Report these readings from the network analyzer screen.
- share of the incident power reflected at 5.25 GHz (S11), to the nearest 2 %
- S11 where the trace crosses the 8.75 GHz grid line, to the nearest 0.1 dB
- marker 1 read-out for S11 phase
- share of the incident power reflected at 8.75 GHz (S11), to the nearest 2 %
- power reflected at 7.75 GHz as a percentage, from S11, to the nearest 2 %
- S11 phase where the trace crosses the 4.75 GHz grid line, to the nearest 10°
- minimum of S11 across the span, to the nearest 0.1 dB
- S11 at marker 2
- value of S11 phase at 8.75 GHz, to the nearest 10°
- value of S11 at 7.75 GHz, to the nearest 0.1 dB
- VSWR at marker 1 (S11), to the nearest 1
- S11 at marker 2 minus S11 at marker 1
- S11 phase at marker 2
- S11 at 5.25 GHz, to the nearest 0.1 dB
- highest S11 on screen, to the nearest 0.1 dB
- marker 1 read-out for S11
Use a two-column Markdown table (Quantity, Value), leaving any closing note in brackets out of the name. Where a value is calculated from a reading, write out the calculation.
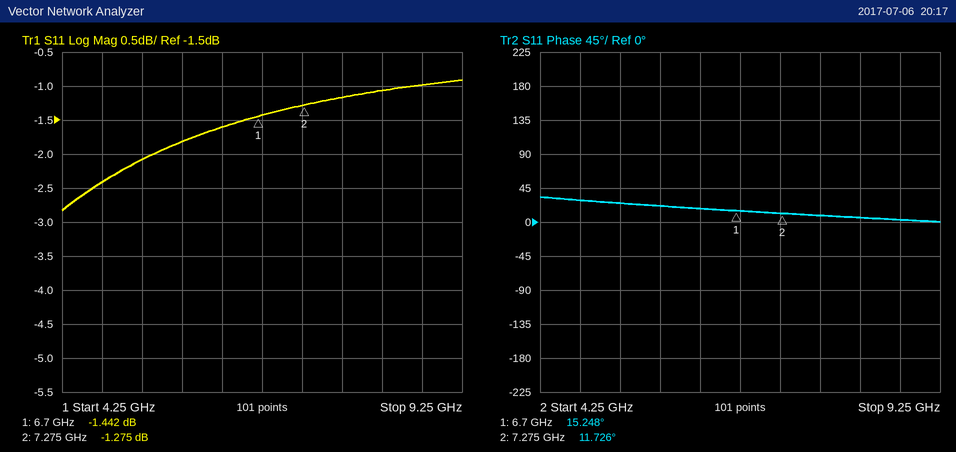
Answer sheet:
| Quantity | Value |
|---|---|
| share of the incident power reflected at 5.25 GHz (S11), to the nearest 2 % | 10^(-2.1/10) ≈ 62 % |
| S11 where the trace crosses the 8.75 GHz grid line, to the nearest 0.1 dB | -1.0 dB |
| marker 1 read-out for S11 phase | 15.248° |
| share of the incident power reflected at 8.75 GHz (S11), to the nearest 2 % | 10^(-1/10) ≈ 79.4 %, so 80 % to the nearest 2 % |
| power reflected at 7.75 GHz as a percentage, from S11, to the nearest 2 % | 10^(-1.2/10) ≈ 76 % |
| S11 phase where the trace crosses the 4.75 GHz grid line, to the nearest 10° | 30° |
| minimum of S11 across the span, to the nearest 0.1 dB | -2.8 dB |
| S11 at marker 2 | -1.275 dB |
| value of S11 phase at 8.75 GHz, to the nearest 10° | 0° |
| value of S11 at 7.75 GHz, to the nearest 0.1 dB | -1.2 dB |
| VSWR at marker 1 (S11), to the nearest 1 | (1 + 0.8470)/(1 − 0.8470) ≈ 12 |
| S11 at marker 2 minus S11 at marker 1 | -1.275 − (-1.442) = 0.167 dB |
| S11 phase at marker 2 | 11.726° |
| S11 at 5.25 GHz, to the nearest 0.1 dB | -2.1 dB |
| highest S11 on screen, to the nearest 0.1 dB | -0.9 dB |
| marker 1 read-out for S11 | -1.442 dB |
